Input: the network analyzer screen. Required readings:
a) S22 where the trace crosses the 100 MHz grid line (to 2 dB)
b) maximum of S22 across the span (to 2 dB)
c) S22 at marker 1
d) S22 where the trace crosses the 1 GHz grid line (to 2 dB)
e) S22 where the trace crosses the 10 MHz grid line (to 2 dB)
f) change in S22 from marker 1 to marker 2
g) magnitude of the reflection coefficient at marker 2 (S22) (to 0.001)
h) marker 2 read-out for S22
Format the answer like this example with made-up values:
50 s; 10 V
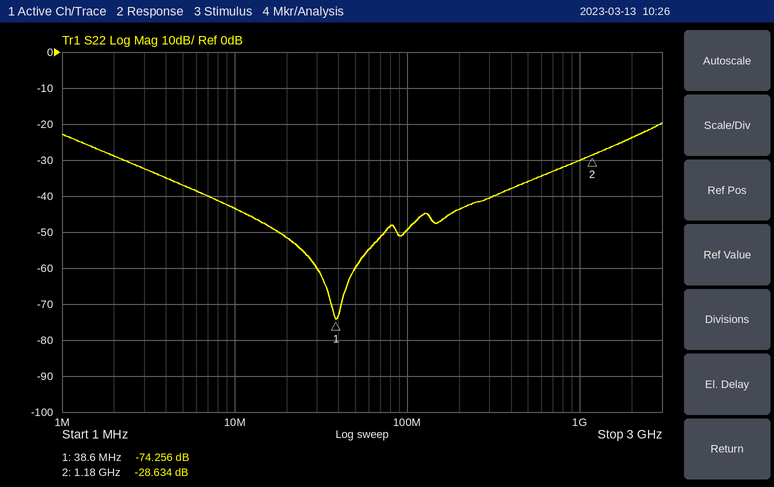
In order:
-50 dB; -20 dB; -74.256 dB; -30 dB; -44 dB; 45.622 dB; 0.037; -28.634 dB
